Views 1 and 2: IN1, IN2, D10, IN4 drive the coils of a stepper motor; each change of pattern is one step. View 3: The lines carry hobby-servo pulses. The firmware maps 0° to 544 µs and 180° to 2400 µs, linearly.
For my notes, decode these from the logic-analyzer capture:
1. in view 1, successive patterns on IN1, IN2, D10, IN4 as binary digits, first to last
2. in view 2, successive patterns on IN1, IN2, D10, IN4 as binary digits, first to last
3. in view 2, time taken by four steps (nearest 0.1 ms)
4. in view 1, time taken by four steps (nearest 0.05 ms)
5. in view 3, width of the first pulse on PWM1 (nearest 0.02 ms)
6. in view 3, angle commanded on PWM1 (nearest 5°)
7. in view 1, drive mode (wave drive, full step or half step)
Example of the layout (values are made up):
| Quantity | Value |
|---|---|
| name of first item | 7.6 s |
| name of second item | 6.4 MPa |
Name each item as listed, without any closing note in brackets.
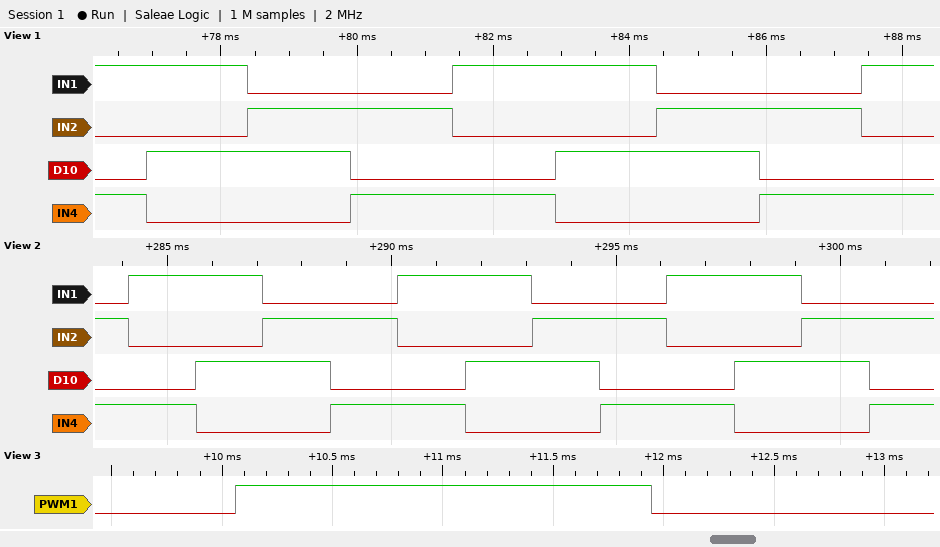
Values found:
| Quantity | Value |
|---|---|
| in view 1, successive patterns on IN1, IN2, D10, IN4 as binary digits, first to last | 1001 1010 0110 0101 1001 1010 0110 0101 1001 |
| in view 2, successive patterns on IN1, IN2, D10, IN4 as binary digits, first to last | 0101 1001 1010 0110 0101 1001 1010 0110 0101 1001 1010 0110 0101 |
| in view 2, time taken by four steps | 6.0 ms |
| in view 1, time taken by four steps | 6.00 ms |
| in view 3, width of the first pulse on PWM1 | 1.88 ms |
| in view 3, angle commanded on PWM1 | 130° |
| in view 1, drive mode | full step |
